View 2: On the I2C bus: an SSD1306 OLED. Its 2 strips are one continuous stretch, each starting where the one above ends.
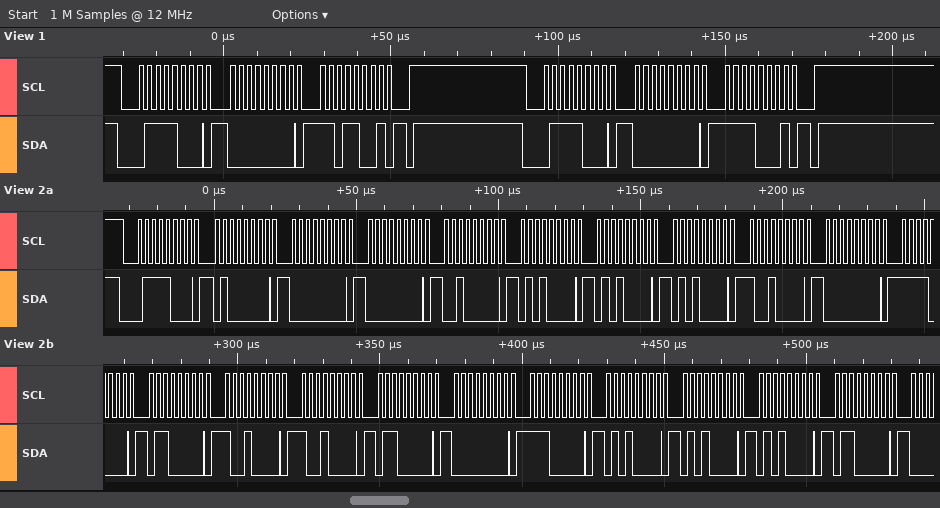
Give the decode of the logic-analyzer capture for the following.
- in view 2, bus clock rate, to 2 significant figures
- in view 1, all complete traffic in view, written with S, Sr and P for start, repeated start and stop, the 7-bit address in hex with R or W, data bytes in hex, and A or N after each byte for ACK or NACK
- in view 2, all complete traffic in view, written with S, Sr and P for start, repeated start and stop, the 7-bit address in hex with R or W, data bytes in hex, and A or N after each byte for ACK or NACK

400 kHz
S 3CW A 00 A D9 A P S 3CW A 00 A F1 A P
S 3CW A 40 A 00 A 00 A 20 A 50 A 50 A 50 A 90 A 00 A F0 A 60 A 90 A 90 A 60 A 00 A E0 A 50 A 50 A 50 A 60 A
